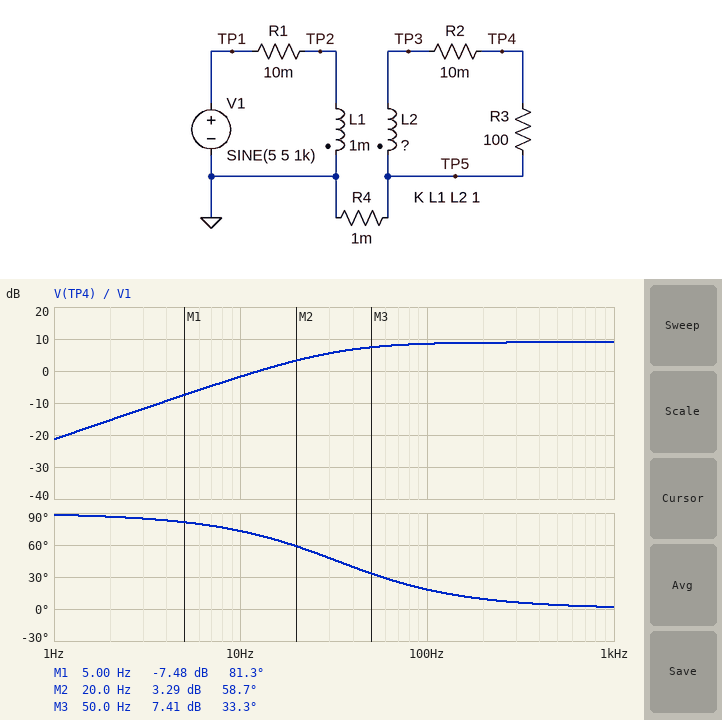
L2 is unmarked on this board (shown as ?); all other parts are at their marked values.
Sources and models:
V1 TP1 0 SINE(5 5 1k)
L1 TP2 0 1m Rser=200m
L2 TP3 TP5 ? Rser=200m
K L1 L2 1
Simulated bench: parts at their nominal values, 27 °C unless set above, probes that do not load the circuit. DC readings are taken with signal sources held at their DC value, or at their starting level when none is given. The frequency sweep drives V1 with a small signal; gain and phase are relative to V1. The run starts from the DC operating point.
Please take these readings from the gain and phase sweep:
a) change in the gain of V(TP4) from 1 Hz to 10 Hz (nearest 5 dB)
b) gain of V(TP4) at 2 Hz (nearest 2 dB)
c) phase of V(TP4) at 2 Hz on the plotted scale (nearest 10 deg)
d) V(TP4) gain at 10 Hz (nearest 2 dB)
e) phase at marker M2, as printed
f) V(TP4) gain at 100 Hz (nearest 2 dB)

20 dB
-16 dB
90 deg
-2 dB
58.7 deg
8 dB
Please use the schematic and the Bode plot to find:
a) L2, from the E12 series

8.2 mH
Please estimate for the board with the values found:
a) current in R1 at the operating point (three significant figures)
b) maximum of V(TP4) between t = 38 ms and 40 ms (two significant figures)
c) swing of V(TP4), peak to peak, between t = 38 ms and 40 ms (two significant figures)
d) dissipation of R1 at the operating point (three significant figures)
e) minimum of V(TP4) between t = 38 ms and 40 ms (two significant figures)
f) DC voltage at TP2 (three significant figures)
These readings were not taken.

23.8 A
14 V
28 V
5.67 W
-14 V
4.76 V
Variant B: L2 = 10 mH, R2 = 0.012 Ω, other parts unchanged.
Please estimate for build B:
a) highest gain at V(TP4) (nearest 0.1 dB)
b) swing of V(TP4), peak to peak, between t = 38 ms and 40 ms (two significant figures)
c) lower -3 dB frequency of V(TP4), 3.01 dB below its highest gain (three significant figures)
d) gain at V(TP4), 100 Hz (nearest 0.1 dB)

9.8 dB
31 V
32.7 Hz
9.4 dB
